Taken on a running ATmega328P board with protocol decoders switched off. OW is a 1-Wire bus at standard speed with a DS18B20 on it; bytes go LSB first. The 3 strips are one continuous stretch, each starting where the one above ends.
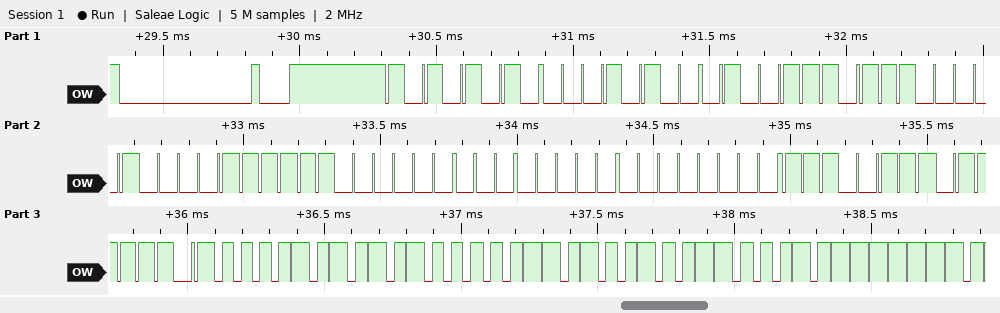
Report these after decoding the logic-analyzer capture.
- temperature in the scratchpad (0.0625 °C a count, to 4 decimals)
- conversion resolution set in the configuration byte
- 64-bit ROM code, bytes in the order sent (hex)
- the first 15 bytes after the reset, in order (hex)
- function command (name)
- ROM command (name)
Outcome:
85.0000 °C
12 bits
28 72 87 F0 03 00 00 E7
55 28 72 87 F0 03 00 00 E7 BE 50 05 4B 46 7F
Read Scratchpad
Match ROM
